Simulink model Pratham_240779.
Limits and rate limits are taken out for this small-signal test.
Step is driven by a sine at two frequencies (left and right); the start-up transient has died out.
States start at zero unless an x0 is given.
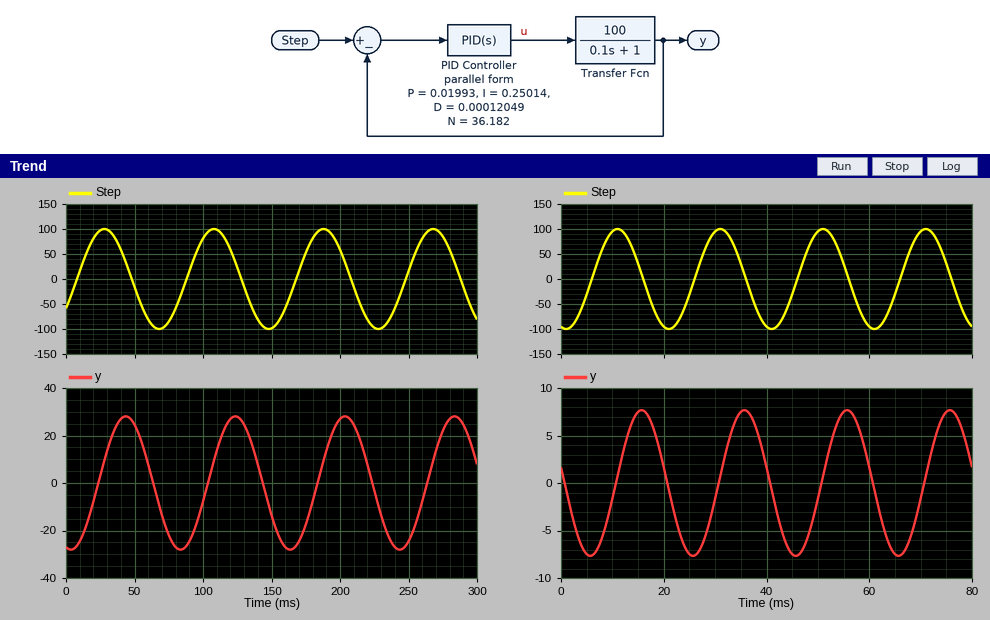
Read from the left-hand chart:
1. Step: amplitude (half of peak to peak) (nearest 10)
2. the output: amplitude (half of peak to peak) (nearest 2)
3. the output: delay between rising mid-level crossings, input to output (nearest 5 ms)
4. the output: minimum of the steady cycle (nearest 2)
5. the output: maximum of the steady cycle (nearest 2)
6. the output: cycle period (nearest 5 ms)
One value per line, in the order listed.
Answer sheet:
100
28
15 ms
-28
28
80 ms
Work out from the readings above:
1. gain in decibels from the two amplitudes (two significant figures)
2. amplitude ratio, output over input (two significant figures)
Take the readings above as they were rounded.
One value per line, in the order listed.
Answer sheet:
-11 dB
0.28
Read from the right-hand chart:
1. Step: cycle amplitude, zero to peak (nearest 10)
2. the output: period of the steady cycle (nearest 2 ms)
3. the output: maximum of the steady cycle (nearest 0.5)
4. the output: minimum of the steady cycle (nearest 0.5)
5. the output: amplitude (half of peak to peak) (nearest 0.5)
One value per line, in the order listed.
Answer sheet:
100
20 ms
7.5
-7.5
7.5
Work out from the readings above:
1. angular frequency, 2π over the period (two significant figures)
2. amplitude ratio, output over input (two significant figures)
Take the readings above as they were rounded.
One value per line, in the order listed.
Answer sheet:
0.31 rad/ms
0.075
